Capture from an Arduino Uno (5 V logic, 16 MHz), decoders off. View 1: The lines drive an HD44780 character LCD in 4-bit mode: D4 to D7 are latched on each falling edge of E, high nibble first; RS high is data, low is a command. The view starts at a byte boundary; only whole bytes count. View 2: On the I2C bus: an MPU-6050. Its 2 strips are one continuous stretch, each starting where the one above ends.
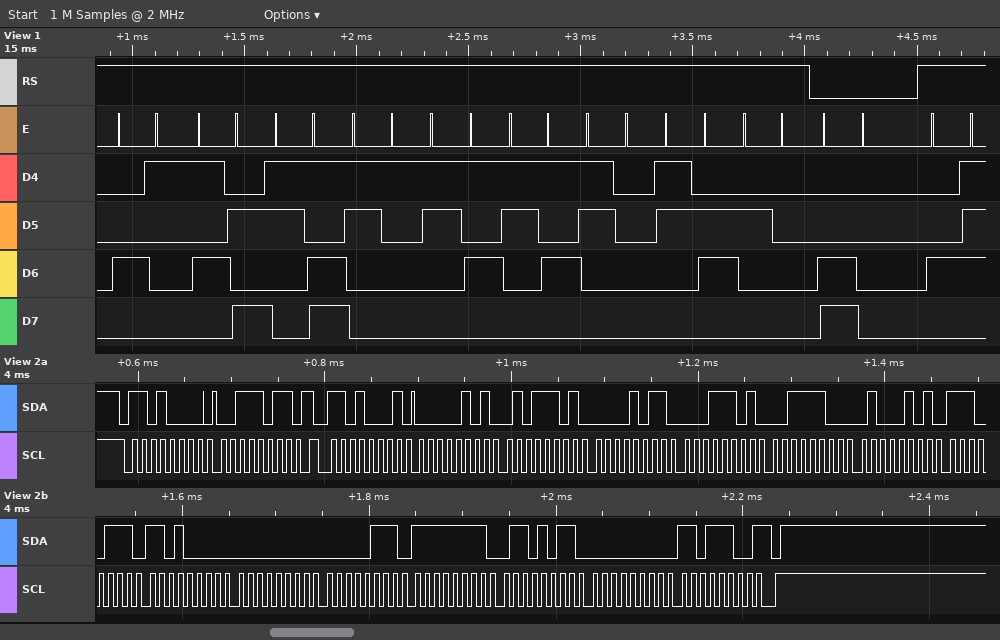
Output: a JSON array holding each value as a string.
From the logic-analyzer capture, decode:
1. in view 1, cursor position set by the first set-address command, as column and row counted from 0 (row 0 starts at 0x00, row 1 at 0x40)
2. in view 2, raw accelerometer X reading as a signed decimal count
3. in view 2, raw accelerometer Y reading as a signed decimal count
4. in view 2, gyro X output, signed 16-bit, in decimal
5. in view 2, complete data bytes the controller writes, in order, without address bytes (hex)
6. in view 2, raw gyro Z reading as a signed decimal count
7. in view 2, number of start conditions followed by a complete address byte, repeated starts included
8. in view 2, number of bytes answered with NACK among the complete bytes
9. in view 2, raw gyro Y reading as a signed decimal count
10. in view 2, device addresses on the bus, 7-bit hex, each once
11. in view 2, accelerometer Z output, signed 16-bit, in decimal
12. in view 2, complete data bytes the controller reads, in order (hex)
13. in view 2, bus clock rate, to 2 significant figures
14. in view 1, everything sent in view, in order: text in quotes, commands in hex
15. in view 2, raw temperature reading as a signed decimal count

["column 0, row 1", "1373", "2845", "7", "3B", "220", "2", "1", "-149", "0x68", "15429", "05 5D 0B 1D 3C 45 E7 D0 00 07 FF 6B 00 DC", "100 kHz", "\"AZ=15506 \" 0xC0 \"G\"", "-6192"]
